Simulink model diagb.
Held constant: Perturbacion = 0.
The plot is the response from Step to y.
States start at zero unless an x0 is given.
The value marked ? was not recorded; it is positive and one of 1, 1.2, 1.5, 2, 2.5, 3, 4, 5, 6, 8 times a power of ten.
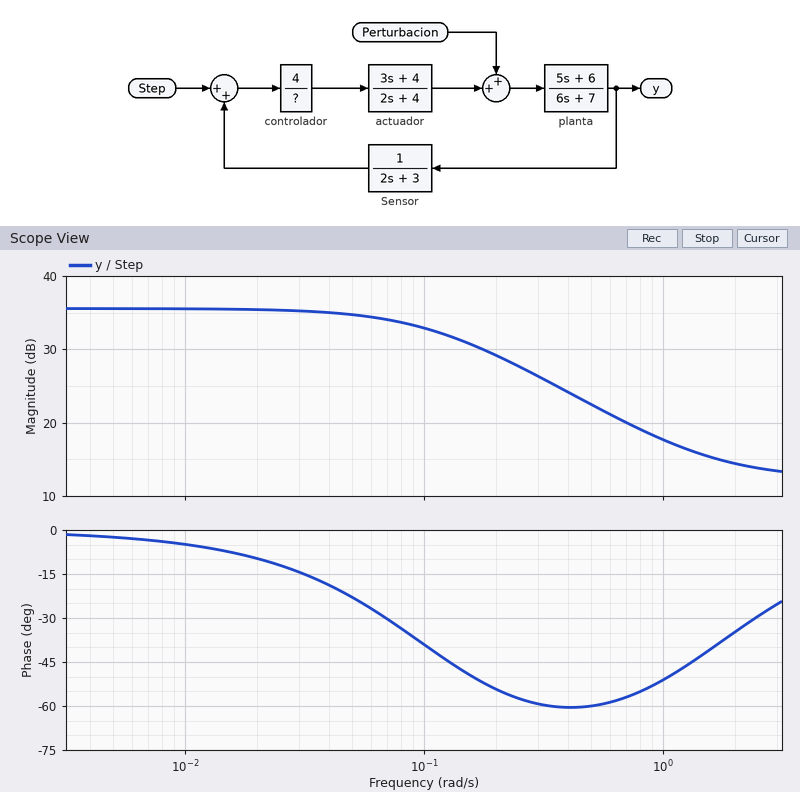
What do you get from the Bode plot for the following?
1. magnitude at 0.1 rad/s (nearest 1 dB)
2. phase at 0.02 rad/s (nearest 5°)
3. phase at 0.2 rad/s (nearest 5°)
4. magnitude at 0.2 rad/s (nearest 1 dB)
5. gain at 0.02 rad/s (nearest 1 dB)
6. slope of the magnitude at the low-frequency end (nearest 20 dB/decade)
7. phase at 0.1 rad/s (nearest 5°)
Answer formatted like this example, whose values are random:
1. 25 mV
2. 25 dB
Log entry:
1. 33 dB
2. -10°
3. -55°
4. 29 dB
5. 35 dB
6. 0 dB/decade
7. -40°
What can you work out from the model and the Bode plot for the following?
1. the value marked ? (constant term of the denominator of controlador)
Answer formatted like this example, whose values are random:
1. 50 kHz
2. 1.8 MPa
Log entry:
1. 1.2
